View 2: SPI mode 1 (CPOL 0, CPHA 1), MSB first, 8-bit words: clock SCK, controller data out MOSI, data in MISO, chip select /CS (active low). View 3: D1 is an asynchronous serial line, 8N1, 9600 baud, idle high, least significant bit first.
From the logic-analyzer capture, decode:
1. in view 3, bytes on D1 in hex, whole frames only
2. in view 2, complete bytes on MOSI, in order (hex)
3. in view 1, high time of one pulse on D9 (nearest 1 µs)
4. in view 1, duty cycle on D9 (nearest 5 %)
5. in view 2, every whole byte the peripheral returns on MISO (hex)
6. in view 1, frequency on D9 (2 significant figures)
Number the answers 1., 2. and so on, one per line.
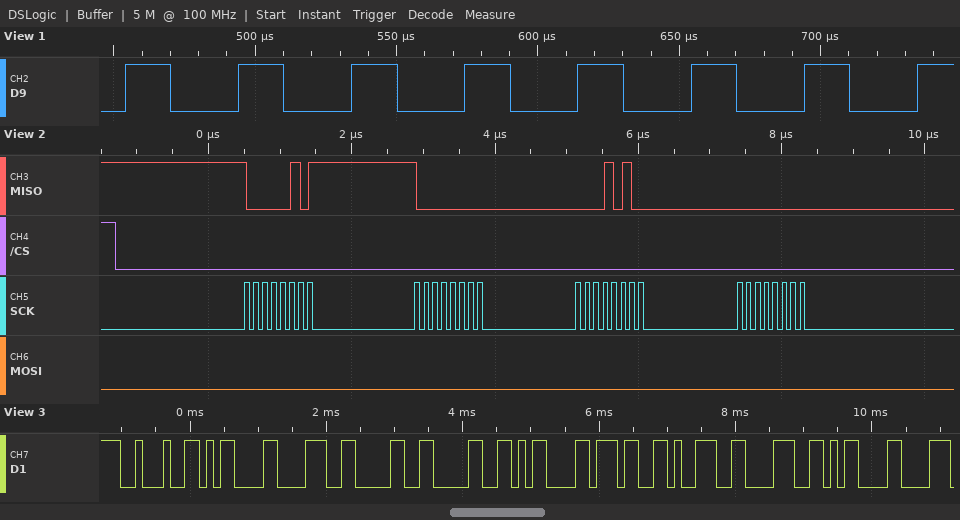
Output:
1. 22 0D 38 30 30 0D 37 39 38 0D
2. 0x00 0x00 0x00 0x00
3. 16 µs
4. 40 %
5. 0x05 0x00 0x14 0x00
6. 25 kHz
